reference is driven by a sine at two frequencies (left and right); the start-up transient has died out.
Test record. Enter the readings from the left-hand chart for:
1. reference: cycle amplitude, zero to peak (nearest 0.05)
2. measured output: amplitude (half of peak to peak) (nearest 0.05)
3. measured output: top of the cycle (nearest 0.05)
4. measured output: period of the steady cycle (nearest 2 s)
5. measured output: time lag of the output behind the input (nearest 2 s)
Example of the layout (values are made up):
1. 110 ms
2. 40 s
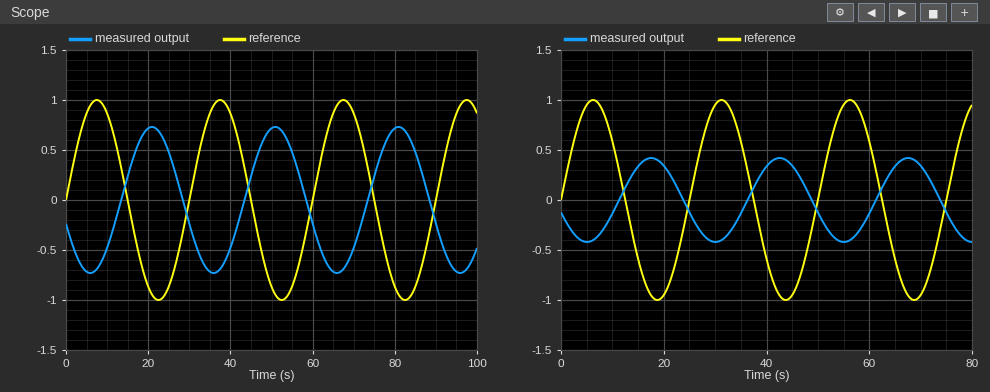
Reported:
1. 1.00
2. 0.75
3. 0.75
4. 30 s
5. 14 s
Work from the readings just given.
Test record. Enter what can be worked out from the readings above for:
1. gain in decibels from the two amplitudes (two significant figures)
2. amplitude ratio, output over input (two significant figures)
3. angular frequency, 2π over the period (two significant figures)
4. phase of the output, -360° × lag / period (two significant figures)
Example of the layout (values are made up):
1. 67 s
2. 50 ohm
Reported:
1. -2.5 dB
2. 0.75
3. 0.21 rad/s
4. -170°
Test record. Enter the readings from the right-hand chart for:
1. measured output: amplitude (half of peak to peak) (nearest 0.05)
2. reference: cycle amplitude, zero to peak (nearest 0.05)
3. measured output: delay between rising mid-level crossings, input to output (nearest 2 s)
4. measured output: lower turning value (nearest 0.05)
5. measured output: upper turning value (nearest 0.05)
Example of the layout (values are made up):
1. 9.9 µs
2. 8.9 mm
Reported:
1. 0.40
2. 1.00
3. 12 s
4. -0.40
5. 0.40
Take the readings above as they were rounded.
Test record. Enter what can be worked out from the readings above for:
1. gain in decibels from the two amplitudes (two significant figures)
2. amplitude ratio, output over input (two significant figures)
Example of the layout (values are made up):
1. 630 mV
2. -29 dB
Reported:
1. -8.0 dB
2. 0.40
